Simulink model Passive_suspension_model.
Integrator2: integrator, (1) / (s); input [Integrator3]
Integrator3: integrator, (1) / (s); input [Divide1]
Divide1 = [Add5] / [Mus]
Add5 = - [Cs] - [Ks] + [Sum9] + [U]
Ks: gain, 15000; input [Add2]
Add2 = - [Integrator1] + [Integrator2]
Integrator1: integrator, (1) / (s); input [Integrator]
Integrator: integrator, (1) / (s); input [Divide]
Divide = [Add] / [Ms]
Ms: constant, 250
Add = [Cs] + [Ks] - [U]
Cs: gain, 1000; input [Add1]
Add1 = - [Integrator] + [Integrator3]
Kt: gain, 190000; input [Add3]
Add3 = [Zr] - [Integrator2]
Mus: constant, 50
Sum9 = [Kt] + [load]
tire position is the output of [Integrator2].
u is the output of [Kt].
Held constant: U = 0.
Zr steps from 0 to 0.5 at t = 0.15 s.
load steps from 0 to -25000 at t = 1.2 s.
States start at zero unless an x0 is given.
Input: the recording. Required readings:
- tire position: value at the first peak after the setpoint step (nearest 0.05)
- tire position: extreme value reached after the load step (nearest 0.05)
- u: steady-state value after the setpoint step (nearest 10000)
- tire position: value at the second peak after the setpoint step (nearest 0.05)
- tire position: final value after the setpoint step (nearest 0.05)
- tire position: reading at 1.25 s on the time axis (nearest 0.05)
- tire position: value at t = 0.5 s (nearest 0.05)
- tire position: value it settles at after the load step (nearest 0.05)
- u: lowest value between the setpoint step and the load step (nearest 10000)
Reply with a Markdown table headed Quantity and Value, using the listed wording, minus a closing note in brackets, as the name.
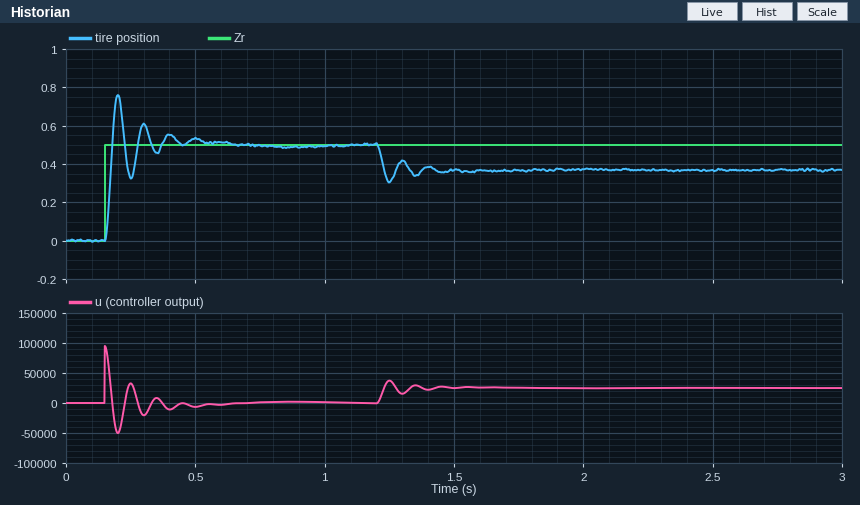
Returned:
| Quantity | Value |
|---|---|
| tire position: value at the first peak after the setpoint step | 0.75 |
| tire position: extreme value reached after the load step | 0.30 |
| u: steady-state value after the setpoint step | 0 |
| tire position: value at the second peak after the setpoint step | 0.60 |
| tire position: final value after the setpoint step | 0.50 |
| tire position: reading at 1.25 s on the time axis | 0.30 |
| tire position: value at t = 0.5 s | 0.55 |
| tire position: value it settles at after the load step | 0.35 |
| u: lowest value between the setpoint step and the load step | -50000 |
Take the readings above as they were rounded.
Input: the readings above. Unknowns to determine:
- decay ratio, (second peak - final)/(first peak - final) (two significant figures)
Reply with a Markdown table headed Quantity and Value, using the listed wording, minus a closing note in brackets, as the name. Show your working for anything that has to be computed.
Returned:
| Quantity | Value |
|---|---|
| decay ratio, (second peak - final)/(first peak - final) | (0.6 - 0.5) / (0.75 - 0.5) = 0.40 |
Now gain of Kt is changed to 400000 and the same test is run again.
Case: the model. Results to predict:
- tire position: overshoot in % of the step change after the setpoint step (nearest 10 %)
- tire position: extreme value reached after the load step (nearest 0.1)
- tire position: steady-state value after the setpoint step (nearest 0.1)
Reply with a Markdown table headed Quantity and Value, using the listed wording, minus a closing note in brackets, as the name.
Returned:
| Quantity | Value |
|---|---|
| tire position: overshoot in % of the step change after the setpoint step | 70 % |
| tire position: extreme value reached after the load step | 0.4 |
| tire position: steady-state value after the setpoint step | 0.5 |
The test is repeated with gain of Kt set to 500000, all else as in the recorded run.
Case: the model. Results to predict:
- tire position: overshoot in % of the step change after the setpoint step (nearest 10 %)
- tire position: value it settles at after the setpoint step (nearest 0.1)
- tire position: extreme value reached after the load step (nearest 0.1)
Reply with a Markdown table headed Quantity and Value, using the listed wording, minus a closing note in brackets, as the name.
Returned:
| Quantity | Value |
|---|---|
| tire position: overshoot in % of the step change after the setpoint step | 70 % |
| tire position: value it settles at after the setpoint step | 0.5 |
| tire position: extreme value reached after the load step | 0.4 |
